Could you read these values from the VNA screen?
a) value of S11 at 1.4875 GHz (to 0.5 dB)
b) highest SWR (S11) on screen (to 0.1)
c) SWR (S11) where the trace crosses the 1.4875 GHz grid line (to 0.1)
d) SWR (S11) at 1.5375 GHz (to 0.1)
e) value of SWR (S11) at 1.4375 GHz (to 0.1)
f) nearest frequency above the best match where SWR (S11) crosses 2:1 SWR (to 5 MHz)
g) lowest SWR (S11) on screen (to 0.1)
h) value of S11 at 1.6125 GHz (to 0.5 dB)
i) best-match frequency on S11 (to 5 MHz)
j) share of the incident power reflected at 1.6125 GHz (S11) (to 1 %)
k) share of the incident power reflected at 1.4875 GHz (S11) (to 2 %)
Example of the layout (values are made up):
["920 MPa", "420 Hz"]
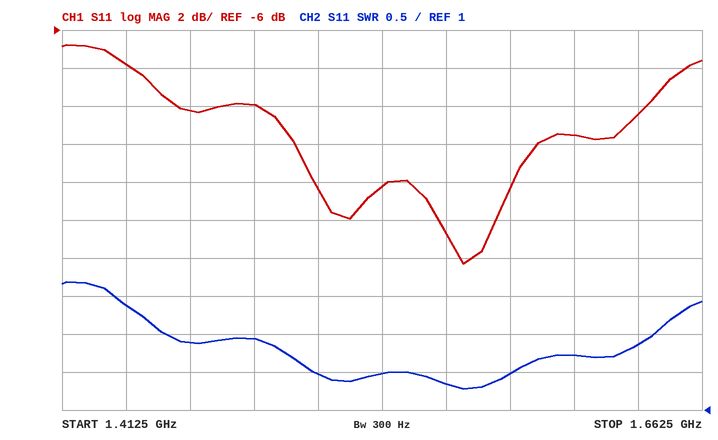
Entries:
["-10.0 dB", "2.7", "1.9", "1.5", "2.4", "1.645 GHz", "1.3", "-11.5 dB", "1.570 GHz", "7 %", "10 %"]
